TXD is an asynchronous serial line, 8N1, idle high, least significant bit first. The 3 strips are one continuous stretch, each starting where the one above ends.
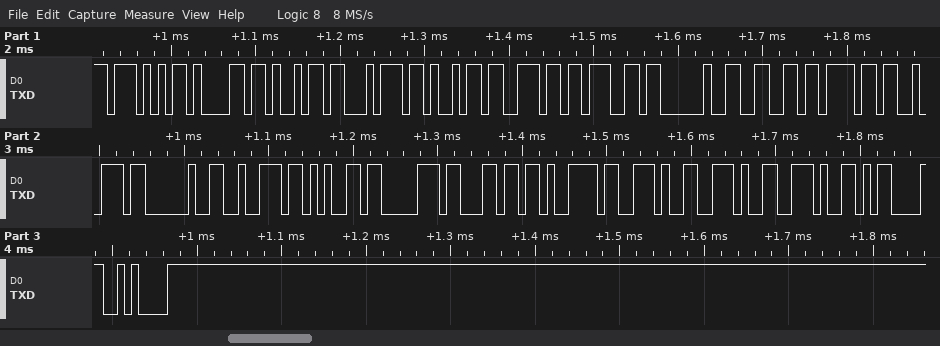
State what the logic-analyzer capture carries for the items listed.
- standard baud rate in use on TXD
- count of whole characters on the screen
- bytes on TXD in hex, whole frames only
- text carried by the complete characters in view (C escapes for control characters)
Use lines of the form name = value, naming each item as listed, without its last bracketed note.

standard baud rate in use on TXD = 115200 baud
count of whole characters on the screen = 22
bytes on TXD in hex, whole frames only = 57 61 69 74 69 6E 67 20 66 6F 72 20 72 65 70 6C 79 2E 2E 2E 0D 0A
text carried by the complete characters in view = "Waiting for reply...\r\n"
